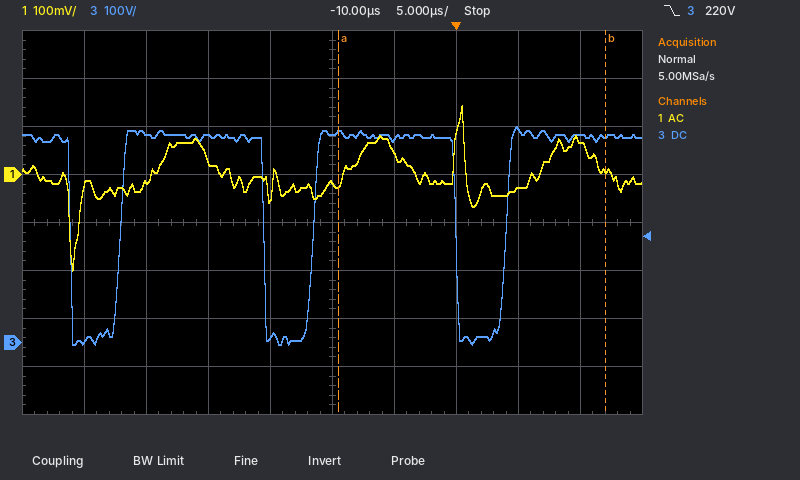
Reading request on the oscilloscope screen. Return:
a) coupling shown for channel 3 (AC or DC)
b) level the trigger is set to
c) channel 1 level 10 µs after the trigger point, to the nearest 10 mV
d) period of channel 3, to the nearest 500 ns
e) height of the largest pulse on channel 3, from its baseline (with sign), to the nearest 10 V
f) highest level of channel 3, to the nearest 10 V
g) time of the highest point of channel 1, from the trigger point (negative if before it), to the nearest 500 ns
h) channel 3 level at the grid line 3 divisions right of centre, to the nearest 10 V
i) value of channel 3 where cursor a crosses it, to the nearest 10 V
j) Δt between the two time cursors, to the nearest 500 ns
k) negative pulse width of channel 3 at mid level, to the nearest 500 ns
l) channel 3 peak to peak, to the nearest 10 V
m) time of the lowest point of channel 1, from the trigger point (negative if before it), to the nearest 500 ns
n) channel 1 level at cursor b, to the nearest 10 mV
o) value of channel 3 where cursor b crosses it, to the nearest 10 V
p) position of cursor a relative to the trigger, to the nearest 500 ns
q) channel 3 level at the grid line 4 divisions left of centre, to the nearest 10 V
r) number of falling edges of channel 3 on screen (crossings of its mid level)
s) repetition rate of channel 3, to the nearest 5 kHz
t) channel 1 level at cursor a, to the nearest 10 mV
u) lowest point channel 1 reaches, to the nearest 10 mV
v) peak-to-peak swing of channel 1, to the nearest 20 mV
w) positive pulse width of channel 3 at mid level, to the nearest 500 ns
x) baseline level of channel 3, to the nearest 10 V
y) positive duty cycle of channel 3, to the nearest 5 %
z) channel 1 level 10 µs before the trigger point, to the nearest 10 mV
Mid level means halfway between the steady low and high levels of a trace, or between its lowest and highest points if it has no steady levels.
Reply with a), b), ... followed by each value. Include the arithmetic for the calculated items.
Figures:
a) DC
b) 220 V
c) 70 mV
d) 15.5 µs
e) 0 V − (430 V) = -430 V
f) 450 V
g) +500 ns
h) 440 V
i) 440 V
j) 21.5 µs
k) 4.0 µs
l) 450 V − (0 V) = 450 V
m) -31.0 µs
n) 10 mV
o) 430 V
p) -9.5 µs
q) 0 V
r) 3
s) 1 / 15.5 µs ≈ 65 kHz
t) -20 mV
u) -200 mV
v) 340 mV
w) 11.5 µs
x) 430 V
y) 11.5 µs / 15.5 µs ≈ 74.2 %, so 75 % to the nearest 5 %
z) -20 mV
